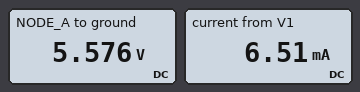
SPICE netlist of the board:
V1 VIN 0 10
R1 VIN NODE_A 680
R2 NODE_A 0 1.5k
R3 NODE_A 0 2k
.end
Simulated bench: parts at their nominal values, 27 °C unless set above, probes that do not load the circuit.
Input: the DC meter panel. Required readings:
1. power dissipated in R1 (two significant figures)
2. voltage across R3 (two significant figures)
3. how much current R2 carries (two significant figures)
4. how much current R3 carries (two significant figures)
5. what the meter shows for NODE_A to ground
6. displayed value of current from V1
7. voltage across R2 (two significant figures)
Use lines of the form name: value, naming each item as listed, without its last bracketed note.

power dissipated in R1: 29 mW
voltage across R3: 5.6 V
how much current R2 carries: 3.7 mA
how much current R3 carries: 2.8 mA
what the meter shows for NODE_A to ground: 5.576 V
displayed value of current from V1: 6.51 mA
voltage across R2: 5.6 V
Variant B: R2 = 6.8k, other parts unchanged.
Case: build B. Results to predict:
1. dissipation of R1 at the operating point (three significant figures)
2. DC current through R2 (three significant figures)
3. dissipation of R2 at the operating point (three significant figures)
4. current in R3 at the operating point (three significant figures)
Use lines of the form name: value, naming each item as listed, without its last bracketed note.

dissipation of R1 at the operating point: 13.7 mW
DC current through R2: 1.02 mA
dissipation of R2 at the operating point: 7.09 mW
current in R3 at the operating point: 3.47 mA
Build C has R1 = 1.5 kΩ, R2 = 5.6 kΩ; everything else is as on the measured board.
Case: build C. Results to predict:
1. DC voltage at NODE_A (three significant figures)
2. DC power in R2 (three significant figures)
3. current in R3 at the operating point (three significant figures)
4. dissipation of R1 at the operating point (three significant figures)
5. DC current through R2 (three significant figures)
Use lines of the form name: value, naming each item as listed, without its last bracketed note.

DC voltage at NODE_A: 4.96 V
DC power in R2: 4.39 mW
current in R3 at the operating point: 2.48 mA
dissipation of R1 at the operating point: 17.0 mW
DC current through R2: 885 µA
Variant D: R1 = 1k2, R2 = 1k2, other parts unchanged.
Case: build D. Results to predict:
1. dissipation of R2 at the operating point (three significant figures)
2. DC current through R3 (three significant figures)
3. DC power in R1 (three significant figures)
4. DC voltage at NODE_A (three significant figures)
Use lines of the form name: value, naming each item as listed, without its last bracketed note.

dissipation of R2 at the operating point: 12.3 mW
DC current through R3: 1.92 mA
DC power in R1: 31.6 mW
DC voltage at NODE_A: 3.85 V
